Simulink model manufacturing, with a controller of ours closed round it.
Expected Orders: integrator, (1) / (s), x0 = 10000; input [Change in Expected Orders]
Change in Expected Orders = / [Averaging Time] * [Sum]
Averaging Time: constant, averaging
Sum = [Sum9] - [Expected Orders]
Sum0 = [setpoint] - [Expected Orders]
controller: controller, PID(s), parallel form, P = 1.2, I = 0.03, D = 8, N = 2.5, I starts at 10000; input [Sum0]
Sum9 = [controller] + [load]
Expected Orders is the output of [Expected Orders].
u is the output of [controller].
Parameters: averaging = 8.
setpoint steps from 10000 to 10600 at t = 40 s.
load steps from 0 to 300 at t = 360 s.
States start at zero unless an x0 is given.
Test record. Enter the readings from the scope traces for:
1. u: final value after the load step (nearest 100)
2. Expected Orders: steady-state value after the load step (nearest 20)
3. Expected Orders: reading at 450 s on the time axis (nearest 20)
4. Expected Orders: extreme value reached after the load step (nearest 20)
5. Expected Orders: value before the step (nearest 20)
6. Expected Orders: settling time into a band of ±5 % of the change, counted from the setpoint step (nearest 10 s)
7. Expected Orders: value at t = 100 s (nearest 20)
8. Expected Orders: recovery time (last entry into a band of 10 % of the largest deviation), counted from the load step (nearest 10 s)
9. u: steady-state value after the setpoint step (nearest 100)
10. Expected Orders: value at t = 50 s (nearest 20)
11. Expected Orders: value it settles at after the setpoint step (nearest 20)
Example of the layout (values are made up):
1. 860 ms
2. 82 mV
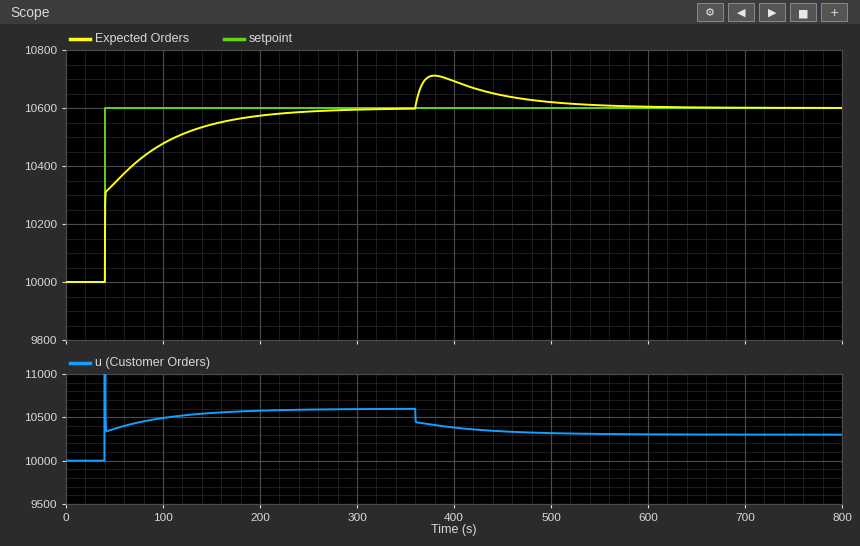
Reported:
1. 10300
2. 10600
3. 10640
4. 10720
5. 10000
6. 150 s
7. 10480
8. 180 s
9. 10600
10. 10340
11. 10600
